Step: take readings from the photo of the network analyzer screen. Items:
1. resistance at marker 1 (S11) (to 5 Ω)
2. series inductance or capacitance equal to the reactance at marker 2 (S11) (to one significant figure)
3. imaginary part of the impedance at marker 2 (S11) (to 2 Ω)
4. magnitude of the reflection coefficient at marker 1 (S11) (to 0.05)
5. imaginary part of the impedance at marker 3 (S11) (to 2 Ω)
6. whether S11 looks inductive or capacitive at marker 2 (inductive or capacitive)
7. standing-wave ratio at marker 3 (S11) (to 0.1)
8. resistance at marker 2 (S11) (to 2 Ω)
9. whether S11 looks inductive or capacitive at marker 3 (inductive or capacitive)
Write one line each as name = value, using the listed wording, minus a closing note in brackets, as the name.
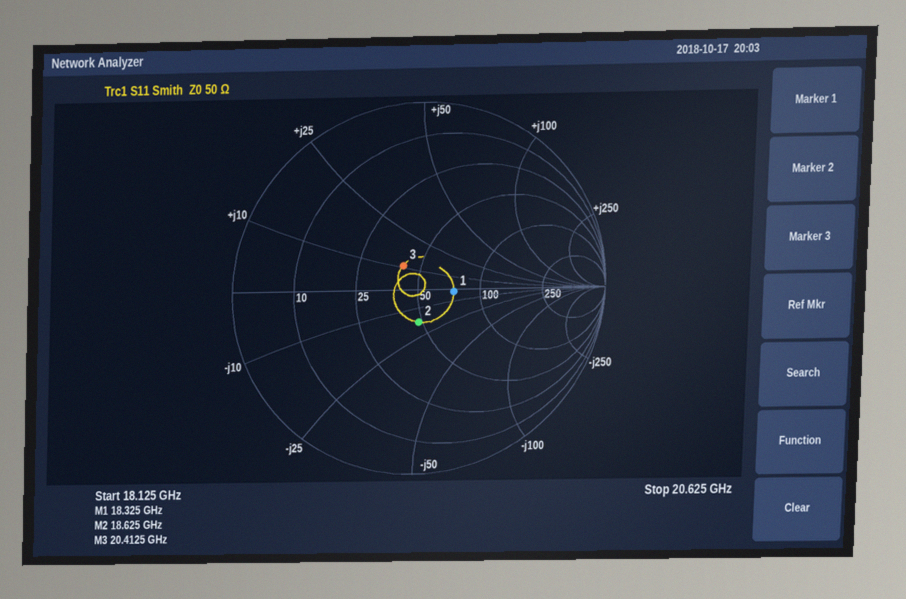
resistance at marker 1 (S11) = 75 Ω
series inductance or capacitance equal to the reactance at marker 2 (S11) = 500 fF
imaginary part of the impedance at marker 2 (S11) = -18 Ω
magnitude of the reflection coefficient at marker 1 (S11) = 0.20
imaginary part of the impedance at marker 3 (S11) = +10 Ω
whether S11 looks inductive or capacitive at marker 2 = capacitive
standing-wave ratio at marker 3 (S11) = 1.4
resistance at marker 2 (S11) = 48 Ω
whether S11 looks inductive or capacitive at marker 3 = inductive
